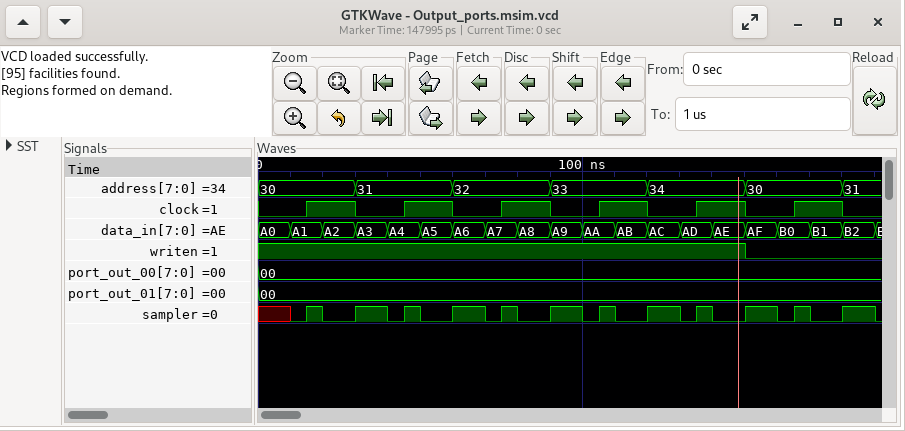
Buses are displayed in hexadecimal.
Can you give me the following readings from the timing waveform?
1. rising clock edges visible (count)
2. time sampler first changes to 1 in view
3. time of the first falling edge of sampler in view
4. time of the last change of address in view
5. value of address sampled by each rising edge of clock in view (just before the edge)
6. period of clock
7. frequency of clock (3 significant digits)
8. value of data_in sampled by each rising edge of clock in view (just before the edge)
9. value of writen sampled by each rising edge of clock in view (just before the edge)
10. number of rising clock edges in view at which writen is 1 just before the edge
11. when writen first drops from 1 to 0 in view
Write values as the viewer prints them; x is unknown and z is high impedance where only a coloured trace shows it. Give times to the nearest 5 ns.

6
15 ns
20 ns
180 ns
30, 31, 32, 33, 34, 30
30 ns
33.3 MHz
A1, A4, A7, AA, AD, B0
1 1 1 1 1 0
5
150 ns
